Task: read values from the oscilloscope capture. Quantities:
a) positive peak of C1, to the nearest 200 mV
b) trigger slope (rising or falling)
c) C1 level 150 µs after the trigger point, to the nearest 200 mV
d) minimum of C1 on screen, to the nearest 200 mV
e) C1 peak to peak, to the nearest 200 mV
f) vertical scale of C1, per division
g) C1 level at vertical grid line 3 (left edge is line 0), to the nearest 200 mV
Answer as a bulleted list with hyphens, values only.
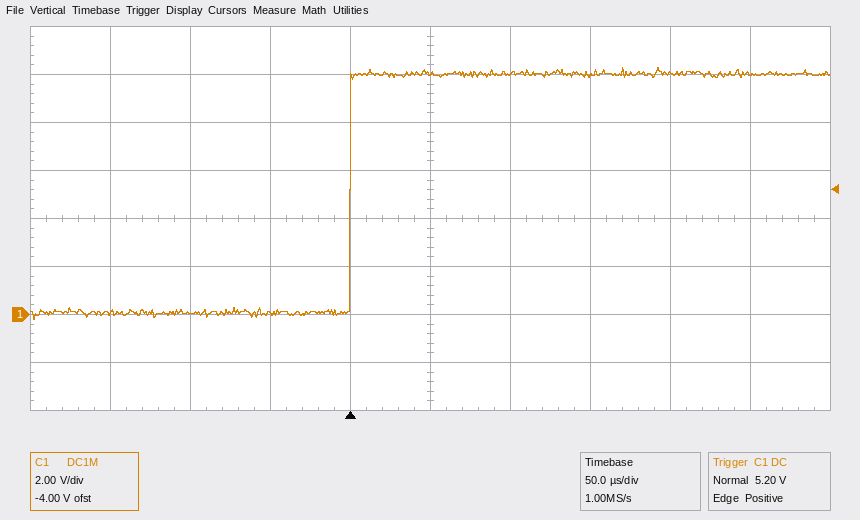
- 10.2 V
- rising
- 10.0 V
- -200 mV
- 10.4 V
- 2 V
- 0.0 V
